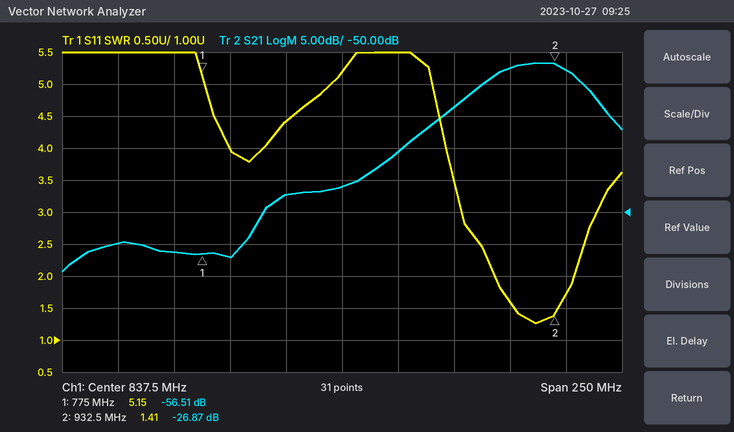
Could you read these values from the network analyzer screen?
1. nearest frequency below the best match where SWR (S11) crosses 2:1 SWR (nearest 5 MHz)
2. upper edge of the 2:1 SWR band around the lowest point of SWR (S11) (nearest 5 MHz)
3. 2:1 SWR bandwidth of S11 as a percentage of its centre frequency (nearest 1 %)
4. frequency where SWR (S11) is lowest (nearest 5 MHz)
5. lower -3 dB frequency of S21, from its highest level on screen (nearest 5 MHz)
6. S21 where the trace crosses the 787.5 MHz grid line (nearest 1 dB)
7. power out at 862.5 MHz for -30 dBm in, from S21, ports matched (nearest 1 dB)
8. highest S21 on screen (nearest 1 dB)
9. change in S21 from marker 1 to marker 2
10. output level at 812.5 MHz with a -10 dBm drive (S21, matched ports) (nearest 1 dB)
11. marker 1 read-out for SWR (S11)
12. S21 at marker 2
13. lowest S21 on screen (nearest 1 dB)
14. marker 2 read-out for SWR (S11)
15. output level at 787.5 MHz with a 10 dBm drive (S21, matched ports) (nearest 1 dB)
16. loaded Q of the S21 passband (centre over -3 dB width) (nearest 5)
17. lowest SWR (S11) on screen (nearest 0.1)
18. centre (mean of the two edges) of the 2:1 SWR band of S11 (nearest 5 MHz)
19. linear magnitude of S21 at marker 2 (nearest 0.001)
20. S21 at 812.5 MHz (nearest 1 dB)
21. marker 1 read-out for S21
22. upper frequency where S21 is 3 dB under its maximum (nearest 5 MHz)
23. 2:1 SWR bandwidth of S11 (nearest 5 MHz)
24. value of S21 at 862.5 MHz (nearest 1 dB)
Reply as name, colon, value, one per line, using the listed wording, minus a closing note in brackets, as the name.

nearest frequency below the best match where SWR (S11) crosses 2:1 SWR: 905 MHz
upper edge of the 2:1 SWR band around the lowest point of SWR (S11): 940 MHz
2:1 SWR bandwidth of S11 as a percentage of its centre frequency: 4 %
frequency where SWR (S11) is lowest: 925 MHz
lower -3 dB frequency of S21, from its highest level on screen: 900 MHz
S21 where the trace crosses the 787.5 MHz grid line: -57 dB
power out at 862.5 MHz for -30 dBm in, from S21, ports matched: -71 dBm
highest S21 on screen: -27 dB
change in S21 from marker 1 to marker 2: 29.64 dB
output level at 812.5 MHz with a -10 dBm drive (S21, matched ports): -57 dBm
marker 1 read-out for SWR: 5.15
S21 at marker 2: -26.87 dB
lowest S21 on screen: -59 dB
marker 2 read-out for SWR: 1.41
output level at 787.5 MHz with a 10 dBm drive (S21, matched ports): -47 dBm
loaded Q of the S21 passband (centre over -3 dB width): 20
lowest SWR (S11) on screen: 1.3
centre (mean of the two edges) of the 2:1 SWR band of S11: 925 MHz
linear magnitude of S21 at marker 2: 0.045
S21 at 812.5 MHz: -47 dB
marker 1 read-out for S21: -56.51 dB
upper frequency where S21 is 3 dB under its maximum: 945 MHz
2:1 SWR bandwidth of S11: 35 MHz
value of S21 at 862.5 MHz: -41 dB
